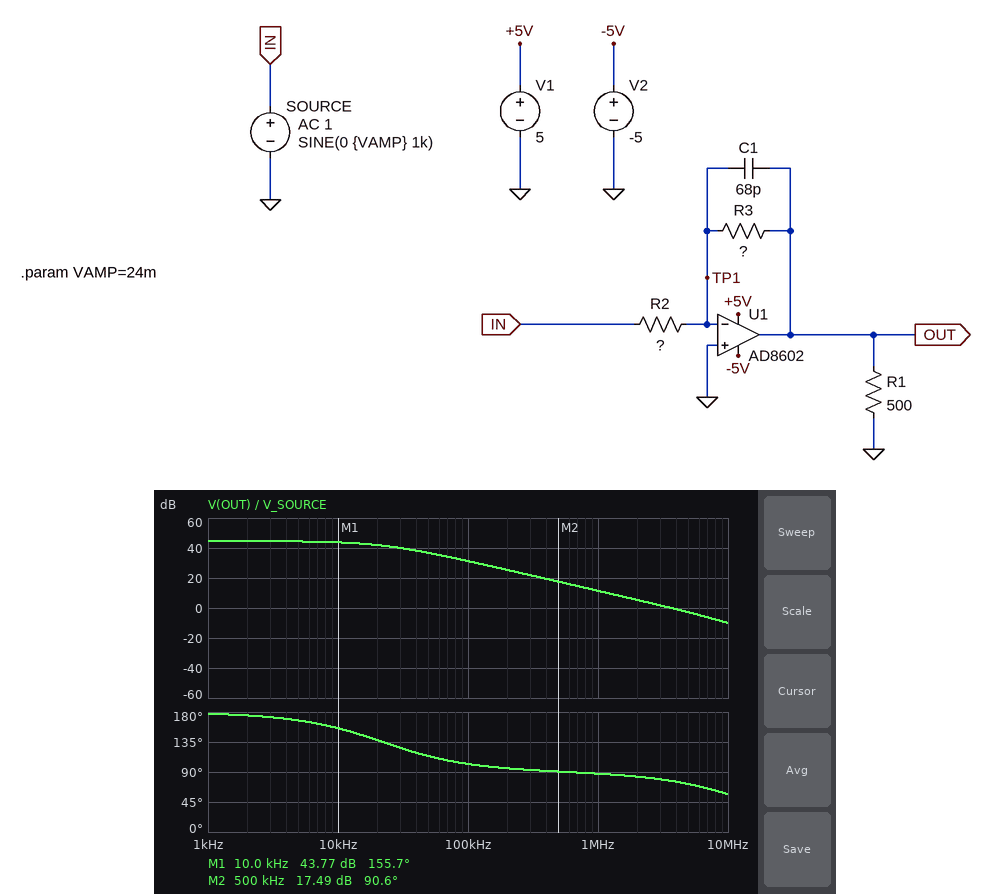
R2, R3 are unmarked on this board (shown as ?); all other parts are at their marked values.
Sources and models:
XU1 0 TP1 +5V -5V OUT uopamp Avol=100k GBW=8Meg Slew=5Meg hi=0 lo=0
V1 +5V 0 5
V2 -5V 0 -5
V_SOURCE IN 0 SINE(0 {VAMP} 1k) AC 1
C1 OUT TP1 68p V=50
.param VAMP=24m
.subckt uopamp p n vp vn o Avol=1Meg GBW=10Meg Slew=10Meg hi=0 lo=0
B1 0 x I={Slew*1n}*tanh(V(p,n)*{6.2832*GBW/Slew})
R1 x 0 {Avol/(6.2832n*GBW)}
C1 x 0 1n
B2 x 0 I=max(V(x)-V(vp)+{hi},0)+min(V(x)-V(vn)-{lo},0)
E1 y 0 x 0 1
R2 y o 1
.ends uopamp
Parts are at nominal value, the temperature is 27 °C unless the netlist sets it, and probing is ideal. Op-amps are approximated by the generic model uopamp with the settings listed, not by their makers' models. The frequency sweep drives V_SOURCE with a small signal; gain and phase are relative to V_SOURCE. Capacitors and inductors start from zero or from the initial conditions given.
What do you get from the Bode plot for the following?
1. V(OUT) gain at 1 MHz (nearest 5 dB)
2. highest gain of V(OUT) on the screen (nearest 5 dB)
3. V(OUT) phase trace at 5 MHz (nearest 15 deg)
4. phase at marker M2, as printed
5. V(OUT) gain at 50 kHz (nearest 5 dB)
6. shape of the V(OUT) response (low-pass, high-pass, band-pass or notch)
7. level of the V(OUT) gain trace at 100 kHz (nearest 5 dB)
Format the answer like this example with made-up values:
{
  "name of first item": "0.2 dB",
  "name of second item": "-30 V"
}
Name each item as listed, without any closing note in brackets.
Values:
{
  "V(OUT) gain at 1 MHz": "10 dB",
  "highest gain of V(OUT) on the screen": "45 dB",
  "V(OUT) phase trace at 5 MHz": "75 deg",
  "phase at marker M2, as printed": "90.6 deg",
  "V(OUT) gain at 50 kHz": "35 dB",
  "shape of the V(OUT) response": "low-pass",
  "level of the V(OUT) gain trace at 100 kHz": "30 dB"
}
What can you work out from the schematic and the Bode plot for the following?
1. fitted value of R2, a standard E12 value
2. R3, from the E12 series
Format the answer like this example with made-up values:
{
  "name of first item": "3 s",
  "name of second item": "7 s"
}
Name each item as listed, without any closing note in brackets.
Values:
{
  "fitted value of R2, a standard E12 value": "330 Ω",
  "R3, from the E12 series": "56 kΩ"
}
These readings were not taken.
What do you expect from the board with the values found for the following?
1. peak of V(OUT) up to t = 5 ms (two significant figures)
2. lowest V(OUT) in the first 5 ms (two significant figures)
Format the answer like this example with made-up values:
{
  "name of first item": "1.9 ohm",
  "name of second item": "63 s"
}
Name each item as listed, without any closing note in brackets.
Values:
{
  "peak of V(OUT) up to t = 5 ms": "4.1 V",
  "lowest V(OUT) in the first 5 ms": "-4.1 V"
}
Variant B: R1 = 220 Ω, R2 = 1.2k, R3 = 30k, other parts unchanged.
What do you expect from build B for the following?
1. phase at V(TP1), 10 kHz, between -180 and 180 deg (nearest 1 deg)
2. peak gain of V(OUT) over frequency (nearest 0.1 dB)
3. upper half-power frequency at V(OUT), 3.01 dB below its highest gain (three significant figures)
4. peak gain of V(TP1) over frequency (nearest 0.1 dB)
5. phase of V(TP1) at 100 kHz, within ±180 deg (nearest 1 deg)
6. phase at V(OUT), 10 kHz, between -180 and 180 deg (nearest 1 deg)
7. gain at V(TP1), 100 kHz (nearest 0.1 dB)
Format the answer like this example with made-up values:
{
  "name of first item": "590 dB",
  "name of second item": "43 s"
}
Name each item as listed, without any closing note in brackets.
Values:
{
  "phase at V(TP1), 10 kHz, between -180 and 180 deg": "80 deg",
  "peak gain of V(OUT) over frequency": "28.0 dB",
  "upper half-power frequency at V(OUT), 3.01 dB below its highest gain": "62.6 kHz",
  "peak gain of V(TP1) over frequency": "-14.2 dB",
  "phase of V(TP1) at 100 kHz, within ±180 deg": "31 deg",
  "phase at V(OUT), 10 kHz, between -180 and 180 deg": "171 deg",
  "gain at V(TP1), 100 kHz": "-15.6 dB"
}
